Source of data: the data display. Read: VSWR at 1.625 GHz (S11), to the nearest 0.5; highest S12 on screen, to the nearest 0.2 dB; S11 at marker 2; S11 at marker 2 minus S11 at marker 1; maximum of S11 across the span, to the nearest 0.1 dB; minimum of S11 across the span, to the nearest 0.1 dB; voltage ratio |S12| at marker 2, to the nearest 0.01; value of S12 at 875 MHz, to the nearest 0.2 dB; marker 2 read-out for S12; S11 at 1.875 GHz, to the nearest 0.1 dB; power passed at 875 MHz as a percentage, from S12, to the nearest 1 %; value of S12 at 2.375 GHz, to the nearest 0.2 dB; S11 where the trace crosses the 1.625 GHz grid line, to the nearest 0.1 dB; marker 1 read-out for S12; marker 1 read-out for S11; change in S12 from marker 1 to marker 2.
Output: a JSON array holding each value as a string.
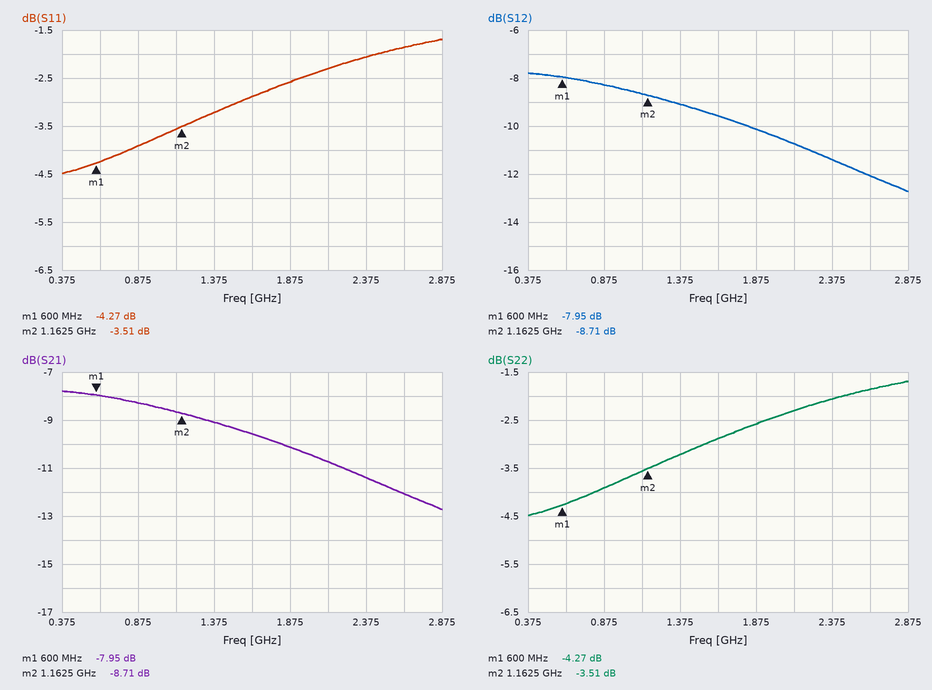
["6.0", "-7.8 dB", "-3.51 dB", "0.76 dB", "-1.7 dB", "-4.5 dB", "0.37", "-8.2 dB", "-8.71 dB", "-2.6 dB", "15 %", "-11.4 dB", "-2.9 dB", "-7.95 dB", "-4.27 dB", "-0.76 dB"]
